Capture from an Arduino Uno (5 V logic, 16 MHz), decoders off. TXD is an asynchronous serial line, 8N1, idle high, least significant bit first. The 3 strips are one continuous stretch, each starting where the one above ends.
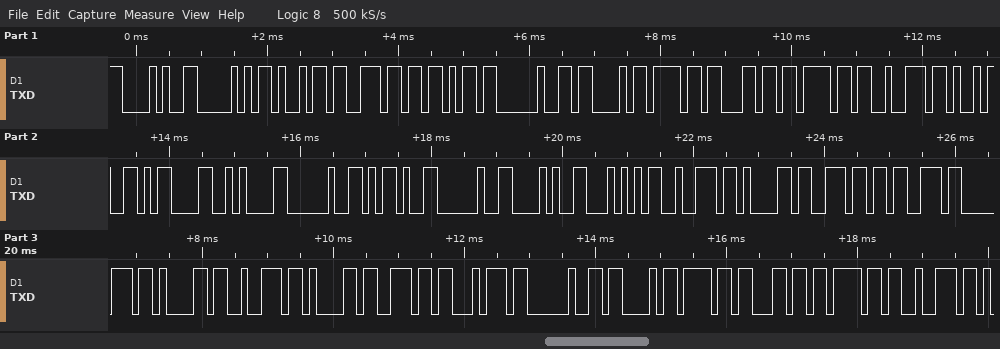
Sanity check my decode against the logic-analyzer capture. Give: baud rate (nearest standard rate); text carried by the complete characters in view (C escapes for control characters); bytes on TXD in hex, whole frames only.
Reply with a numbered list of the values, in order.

1. 9600 baud
2. "(Pink Color)\r\n - (Transparant Color"
3. 28 50 69 6E 6B 20 43 6F 6C 6F 72 29 0D 0A 20 2D 20 28 54 72 61 6E 73 70 61 72 61 6E 74 20 43 6F 6C 6F 72
